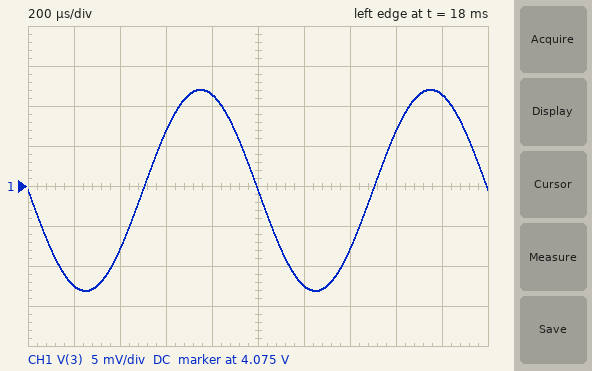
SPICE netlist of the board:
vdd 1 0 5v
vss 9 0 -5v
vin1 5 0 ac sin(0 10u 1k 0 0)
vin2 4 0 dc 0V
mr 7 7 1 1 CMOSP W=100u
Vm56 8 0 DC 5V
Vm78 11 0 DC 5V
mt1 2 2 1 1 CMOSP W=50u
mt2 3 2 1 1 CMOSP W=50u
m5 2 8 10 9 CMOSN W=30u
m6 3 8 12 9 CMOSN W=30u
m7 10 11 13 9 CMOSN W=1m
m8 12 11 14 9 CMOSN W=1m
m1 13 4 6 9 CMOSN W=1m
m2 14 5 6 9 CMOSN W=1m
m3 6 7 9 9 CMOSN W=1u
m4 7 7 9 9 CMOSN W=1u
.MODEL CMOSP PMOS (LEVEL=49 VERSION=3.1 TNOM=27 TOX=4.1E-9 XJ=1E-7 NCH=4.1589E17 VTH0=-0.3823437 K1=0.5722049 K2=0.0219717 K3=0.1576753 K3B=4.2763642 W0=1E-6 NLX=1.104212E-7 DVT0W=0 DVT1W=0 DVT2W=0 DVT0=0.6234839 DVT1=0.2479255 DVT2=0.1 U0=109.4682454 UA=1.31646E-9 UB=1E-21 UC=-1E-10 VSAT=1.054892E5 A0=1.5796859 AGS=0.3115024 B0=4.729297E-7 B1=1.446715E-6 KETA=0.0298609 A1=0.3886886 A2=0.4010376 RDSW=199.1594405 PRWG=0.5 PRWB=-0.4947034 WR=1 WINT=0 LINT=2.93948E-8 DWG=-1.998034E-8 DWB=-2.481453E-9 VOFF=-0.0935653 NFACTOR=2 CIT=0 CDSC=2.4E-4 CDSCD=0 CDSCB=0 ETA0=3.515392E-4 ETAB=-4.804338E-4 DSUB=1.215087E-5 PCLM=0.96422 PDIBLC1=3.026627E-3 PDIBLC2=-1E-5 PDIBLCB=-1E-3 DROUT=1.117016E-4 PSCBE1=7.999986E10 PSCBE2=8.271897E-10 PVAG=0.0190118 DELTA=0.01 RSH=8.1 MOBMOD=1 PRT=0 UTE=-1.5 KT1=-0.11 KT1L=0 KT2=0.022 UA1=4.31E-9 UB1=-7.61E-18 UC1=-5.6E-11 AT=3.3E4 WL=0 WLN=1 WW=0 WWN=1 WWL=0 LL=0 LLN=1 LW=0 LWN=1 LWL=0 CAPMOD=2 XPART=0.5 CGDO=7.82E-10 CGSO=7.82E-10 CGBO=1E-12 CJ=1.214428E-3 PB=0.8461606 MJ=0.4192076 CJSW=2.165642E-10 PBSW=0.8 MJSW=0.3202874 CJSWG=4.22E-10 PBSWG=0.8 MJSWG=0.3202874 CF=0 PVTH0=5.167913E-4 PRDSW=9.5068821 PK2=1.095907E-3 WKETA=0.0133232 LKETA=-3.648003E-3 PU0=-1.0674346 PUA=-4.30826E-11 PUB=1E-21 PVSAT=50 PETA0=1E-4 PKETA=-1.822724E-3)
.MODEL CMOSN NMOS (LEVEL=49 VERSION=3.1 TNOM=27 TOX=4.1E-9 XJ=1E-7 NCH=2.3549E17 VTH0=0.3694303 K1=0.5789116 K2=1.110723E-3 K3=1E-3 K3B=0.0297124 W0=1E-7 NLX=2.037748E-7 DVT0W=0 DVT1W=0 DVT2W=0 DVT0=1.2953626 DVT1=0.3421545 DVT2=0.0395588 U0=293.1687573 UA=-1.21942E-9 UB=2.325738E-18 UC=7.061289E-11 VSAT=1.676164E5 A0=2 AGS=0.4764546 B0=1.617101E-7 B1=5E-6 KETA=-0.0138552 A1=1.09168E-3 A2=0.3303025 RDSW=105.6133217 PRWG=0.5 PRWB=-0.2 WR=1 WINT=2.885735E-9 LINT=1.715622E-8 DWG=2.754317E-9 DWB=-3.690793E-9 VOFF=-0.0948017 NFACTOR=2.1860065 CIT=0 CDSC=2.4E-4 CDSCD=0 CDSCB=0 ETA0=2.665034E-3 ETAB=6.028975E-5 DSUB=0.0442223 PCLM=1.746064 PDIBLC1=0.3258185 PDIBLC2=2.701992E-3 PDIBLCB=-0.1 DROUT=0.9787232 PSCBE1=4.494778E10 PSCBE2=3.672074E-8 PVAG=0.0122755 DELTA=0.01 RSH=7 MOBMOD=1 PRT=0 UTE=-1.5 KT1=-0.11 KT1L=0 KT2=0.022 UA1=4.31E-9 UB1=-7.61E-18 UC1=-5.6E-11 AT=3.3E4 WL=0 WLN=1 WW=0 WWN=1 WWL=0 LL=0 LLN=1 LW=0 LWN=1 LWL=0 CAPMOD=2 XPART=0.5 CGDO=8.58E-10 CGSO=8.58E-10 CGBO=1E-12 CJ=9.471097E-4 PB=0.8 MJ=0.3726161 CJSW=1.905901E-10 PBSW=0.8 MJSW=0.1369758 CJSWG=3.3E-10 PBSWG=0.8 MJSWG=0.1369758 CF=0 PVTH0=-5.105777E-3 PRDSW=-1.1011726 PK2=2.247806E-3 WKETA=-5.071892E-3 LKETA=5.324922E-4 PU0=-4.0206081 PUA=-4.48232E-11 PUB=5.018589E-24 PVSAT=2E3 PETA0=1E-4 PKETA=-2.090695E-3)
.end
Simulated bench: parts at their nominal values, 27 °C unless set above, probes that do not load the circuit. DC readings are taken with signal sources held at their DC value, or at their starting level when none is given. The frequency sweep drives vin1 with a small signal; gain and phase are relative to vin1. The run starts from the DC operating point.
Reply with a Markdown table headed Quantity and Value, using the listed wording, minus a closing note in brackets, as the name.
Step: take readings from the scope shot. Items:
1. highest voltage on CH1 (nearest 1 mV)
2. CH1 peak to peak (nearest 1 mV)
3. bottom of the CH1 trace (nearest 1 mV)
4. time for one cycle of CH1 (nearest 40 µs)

| Quantity | Value |
|---|---|
| highest voltage on CH1 | 4.087 V |
| CH1 peak to peak | 25 mV |
| bottom of the CH1 trace | 4.062 V |
| time for one cycle of CH1 | 1.00 ms |
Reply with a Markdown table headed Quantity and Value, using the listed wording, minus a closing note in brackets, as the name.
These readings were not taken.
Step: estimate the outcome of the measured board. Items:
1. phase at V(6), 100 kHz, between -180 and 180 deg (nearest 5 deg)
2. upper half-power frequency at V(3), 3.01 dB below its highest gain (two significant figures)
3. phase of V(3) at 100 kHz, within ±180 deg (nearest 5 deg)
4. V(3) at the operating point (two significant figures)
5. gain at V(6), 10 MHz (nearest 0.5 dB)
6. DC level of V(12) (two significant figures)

| Quantity | Value |
|---|---|
| phase at V(6), 100 kHz, between -180 and 180 deg | 0 deg |
| upper half-power frequency at V(3), 3.01 dB below its highest gain | 500 kHz |
| phase of V(3) at 100 kHz, within ±180 deg | 165 deg |
| V(3) at the operating point | 4.1 V |
| gain at V(6), 10 MHz | -7.0 dB |
| DC level of V(12) | 3.1 V |
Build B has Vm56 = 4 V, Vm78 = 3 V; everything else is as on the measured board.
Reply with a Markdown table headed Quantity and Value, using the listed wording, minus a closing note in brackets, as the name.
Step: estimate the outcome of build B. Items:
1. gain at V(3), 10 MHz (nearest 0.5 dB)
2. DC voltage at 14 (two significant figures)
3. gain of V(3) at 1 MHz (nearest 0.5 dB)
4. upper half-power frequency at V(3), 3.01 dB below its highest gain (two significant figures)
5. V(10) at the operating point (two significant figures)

| Quantity | Value |
|---|---|
| gain at V(3), 10 MHz | 45.5 dB |
| DC voltage at 14 | 1.6 V |
| gain of V(3) at 1 MHz | 60.5 dB |
| upper half-power frequency at V(3), 3.01 dB below its highest gain | 1.5 MHz |
| V(10) at the operating point | 2.2 V |
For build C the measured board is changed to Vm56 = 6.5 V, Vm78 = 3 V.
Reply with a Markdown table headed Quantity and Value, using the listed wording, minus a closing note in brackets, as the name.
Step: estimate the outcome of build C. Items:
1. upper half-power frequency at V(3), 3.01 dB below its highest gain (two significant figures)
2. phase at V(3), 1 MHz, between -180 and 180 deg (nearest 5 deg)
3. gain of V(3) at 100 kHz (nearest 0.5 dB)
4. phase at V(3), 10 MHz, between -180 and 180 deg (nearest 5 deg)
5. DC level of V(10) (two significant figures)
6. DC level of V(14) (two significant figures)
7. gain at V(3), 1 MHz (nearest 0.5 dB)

| Quantity | Value |
|---|---|
| upper half-power frequency at V(3), 3.01 dB below its highest gain | 91 kHz |
| phase at V(3), 1 MHz, between -180 and 180 deg | 85 deg |
| gain of V(3) at 100 kHz | 58.5 dB |
| phase at V(3), 10 MHz, between -180 and 180 deg | 10 deg |
| DC level of V(10) | 4.0 V |
| DC level of V(14) | 1.6 V |
| gain at V(3), 1 MHz | 41.0 dB |
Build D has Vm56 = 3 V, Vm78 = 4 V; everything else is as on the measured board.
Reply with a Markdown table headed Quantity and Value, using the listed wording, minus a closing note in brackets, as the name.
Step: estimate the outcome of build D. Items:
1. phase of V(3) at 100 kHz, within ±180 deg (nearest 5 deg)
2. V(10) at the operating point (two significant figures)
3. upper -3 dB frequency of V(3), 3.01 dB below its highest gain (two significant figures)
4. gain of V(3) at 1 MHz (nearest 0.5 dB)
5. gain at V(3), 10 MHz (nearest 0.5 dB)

| Quantity | Value |
|---|---|
| phase of V(3) at 100 kHz, within ±180 deg | 170 deg |
| V(10) at the operating point | 1.3 V |
| upper -3 dB frequency of V(3), 3.01 dB below its highest gain | 560 kHz |
| gain of V(3) at 1 MHz | 55.5 dB |
| gain at V(3), 10 MHz | 28.5 dB |
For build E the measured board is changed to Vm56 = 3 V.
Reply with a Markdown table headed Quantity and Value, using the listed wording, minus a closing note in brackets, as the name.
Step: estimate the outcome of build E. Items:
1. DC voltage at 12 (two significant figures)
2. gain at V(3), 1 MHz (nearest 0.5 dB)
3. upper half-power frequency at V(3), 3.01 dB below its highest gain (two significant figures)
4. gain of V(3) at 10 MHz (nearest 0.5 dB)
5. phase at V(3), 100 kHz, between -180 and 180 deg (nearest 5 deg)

| Quantity | Value |
|---|---|
| DC voltage at 12 | 1.3 V |
| gain at V(3), 1 MHz | 55.5 dB |
| upper half-power frequency at V(3), 3.01 dB below its highest gain | 560 kHz |
| gain of V(3) at 10 MHz | 28.5 dB |
| phase at V(3), 100 kHz, between -180 and 180 deg | 170 deg |
